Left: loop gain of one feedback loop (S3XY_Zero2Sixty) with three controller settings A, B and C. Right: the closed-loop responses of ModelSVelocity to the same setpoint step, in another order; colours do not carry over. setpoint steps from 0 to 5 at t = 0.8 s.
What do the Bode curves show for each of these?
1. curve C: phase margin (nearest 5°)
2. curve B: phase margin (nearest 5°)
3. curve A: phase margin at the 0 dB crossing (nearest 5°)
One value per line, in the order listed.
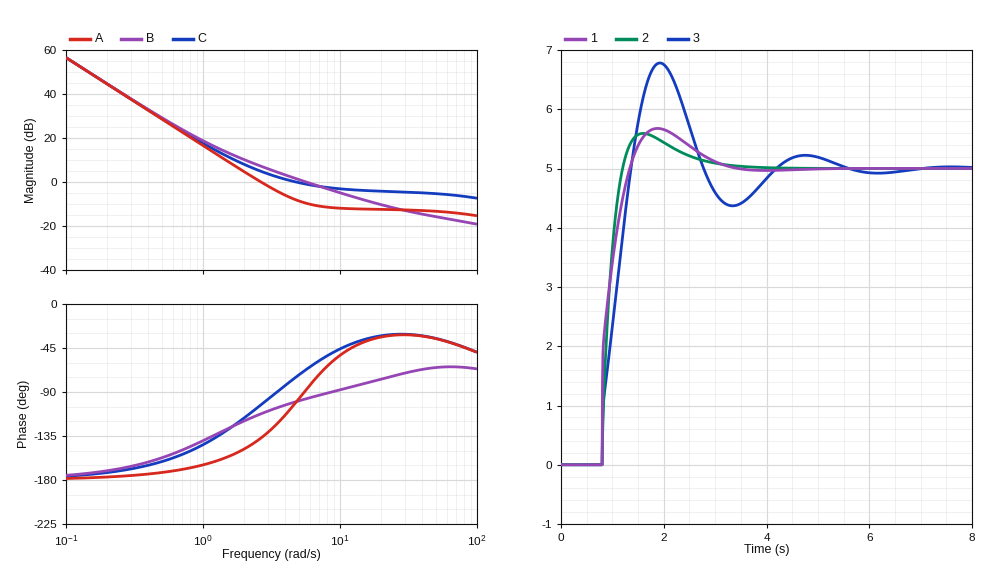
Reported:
105°
85°
45°
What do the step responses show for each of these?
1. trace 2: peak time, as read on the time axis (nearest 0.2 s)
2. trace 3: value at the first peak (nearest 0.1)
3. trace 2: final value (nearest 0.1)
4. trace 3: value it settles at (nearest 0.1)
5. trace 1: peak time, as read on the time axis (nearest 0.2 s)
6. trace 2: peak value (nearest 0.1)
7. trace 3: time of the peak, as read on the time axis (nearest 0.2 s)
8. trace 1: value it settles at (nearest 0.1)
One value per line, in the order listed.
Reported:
1.6 s
6.8
5.0
5.0
1.8 s
5.6
2.0 s
5.0
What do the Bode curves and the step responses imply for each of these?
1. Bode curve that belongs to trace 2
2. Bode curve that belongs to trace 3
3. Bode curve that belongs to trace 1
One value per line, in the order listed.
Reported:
B
A
C
